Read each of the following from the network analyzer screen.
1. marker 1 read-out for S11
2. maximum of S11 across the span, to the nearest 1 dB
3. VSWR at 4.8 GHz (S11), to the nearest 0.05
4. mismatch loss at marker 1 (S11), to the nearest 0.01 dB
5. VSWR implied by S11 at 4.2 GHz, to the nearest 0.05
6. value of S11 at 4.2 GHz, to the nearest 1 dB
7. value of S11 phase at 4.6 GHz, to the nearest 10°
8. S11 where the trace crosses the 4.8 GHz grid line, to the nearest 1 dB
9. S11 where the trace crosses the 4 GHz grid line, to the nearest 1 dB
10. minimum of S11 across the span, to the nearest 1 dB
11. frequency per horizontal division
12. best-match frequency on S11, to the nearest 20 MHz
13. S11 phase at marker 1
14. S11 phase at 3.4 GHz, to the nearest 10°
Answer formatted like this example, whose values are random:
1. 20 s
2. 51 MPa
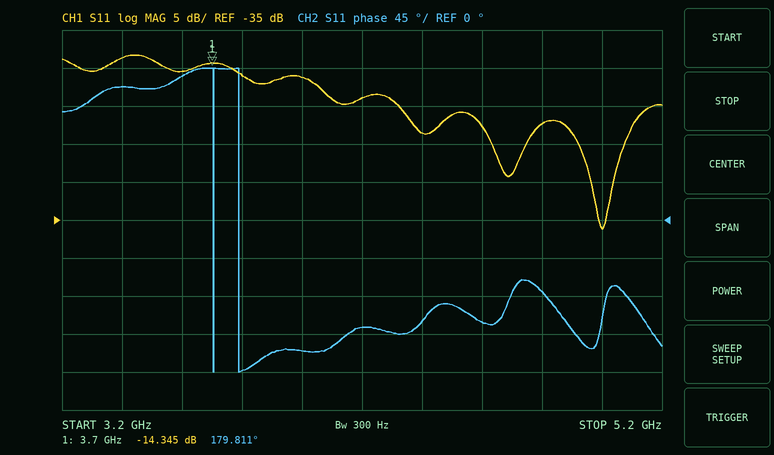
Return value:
1. -14.345 dB
2. -13 dB
3. 1.15
4. 0.16 dB
5. 1.25
6. -19 dB
7. -120°
8. -22 dB
9. -16 dB
10. -36 dB
11. 200 MHz
12. 5.00 GHz
13. 179.811°
14. 160°
